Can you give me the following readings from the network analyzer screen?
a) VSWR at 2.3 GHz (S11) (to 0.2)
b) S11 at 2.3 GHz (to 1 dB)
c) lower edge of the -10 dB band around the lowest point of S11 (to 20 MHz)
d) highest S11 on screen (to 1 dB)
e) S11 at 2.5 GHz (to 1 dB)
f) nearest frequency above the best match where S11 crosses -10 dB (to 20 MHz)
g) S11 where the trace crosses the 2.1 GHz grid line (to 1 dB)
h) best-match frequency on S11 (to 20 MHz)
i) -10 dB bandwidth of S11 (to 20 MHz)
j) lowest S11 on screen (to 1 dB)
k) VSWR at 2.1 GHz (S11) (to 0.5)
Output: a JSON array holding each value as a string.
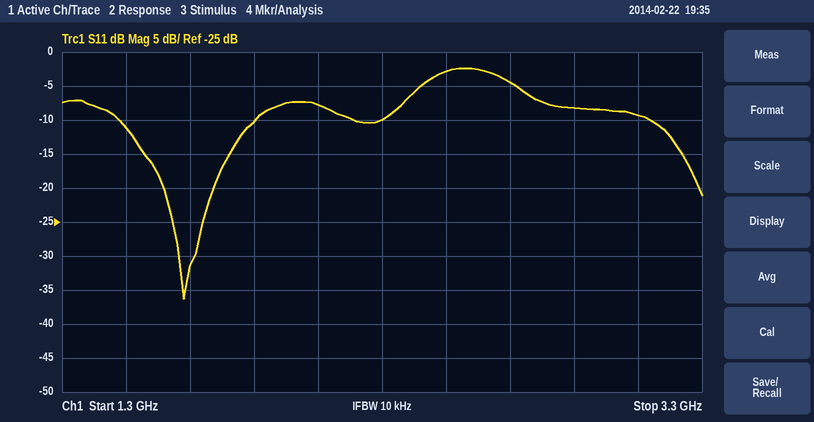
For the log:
["2.0", "-10 dB", "1.48 GHz", "-2 dB", "-3 dB", "1.90 GHz", "-8 dB", "1.68 GHz", "420 MHz", "-36 dB", "2.5"]
